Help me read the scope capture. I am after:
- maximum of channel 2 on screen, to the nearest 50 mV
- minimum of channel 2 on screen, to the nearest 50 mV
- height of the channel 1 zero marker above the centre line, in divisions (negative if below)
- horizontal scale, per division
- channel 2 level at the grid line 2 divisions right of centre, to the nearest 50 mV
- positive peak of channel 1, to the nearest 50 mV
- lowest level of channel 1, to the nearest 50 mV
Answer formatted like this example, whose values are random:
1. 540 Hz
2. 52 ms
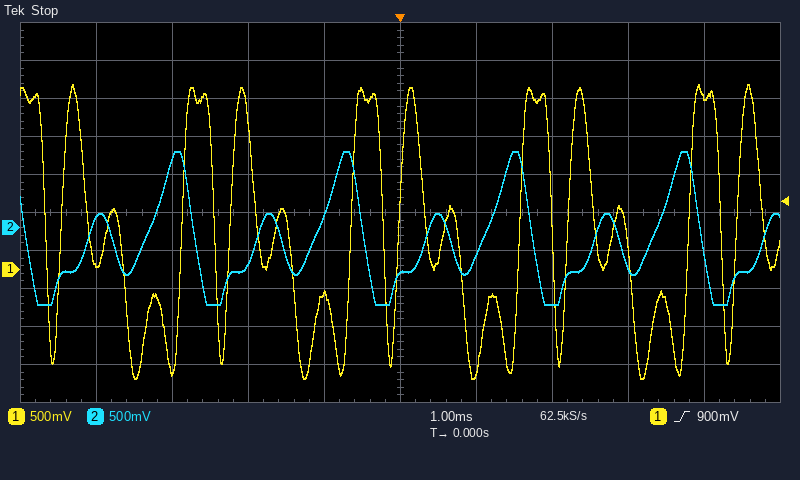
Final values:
1. 1.00 V
2. -1.00 V
3. -1.5 div
4. 1 ms
5. -1.00 V
6. 2.45 V
7. -1.45 V
